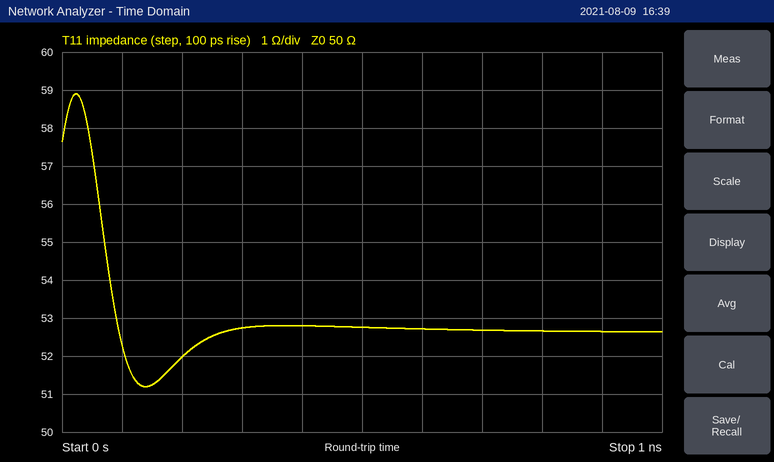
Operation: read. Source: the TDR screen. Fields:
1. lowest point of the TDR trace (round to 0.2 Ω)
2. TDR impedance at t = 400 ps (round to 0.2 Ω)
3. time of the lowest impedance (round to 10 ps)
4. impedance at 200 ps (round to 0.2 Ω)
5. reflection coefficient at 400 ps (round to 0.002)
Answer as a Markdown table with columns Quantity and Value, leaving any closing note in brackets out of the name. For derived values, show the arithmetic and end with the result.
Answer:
| Quantity | Value |
|---|---|
| lowest point of the TDR trace | 51.2 Ω |
| TDR impedance at t = 400 ps | 52.8 Ω |
| time of the lowest impedance | 140 ps |
| impedance at 200 ps | 52.0 Ω |
| reflection coefficient at 400 ps | (52.8 − 50)/(52.8 + 50) ≈ +0.0272, so +0.028 to the nearest 0.002 |
